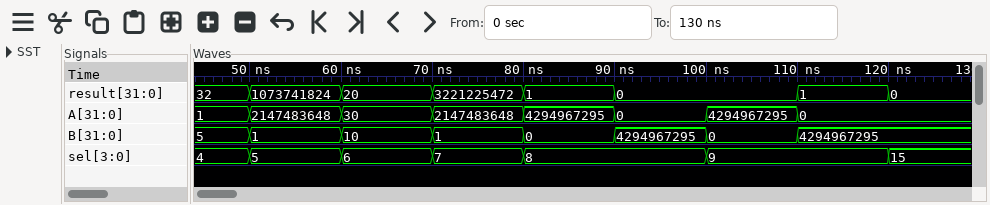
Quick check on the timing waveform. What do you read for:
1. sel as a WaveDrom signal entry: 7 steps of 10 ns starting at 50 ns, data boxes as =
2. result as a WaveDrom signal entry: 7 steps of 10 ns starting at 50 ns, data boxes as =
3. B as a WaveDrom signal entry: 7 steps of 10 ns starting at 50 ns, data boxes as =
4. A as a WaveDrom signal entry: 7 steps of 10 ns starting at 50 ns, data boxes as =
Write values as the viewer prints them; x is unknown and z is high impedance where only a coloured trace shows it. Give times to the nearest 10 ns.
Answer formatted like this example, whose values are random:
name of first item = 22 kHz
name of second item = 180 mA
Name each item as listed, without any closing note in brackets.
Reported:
sel as a WaveDrom signal entry: 7 steps of 10 ns starting at 50 ns, data boxes as = = {name: 'sel', wave: '====.=.', data: '5 6 7 8 9'}
result as a WaveDrom signal entry: 7 steps of 10 ns starting at 50 ns, data boxes as = = {name: 'result', wave: '=====.=', data: '1073741824 20 3221225472 1 0 1'}
B as a WaveDrom signal entry: 7 steps of 10 ns starting at 50 ns, data boxes as = = {name: 'B', wave: '=======', data: '1 10 1 0 4294967295 0 4294967295'}
A as a WaveDrom signal entry: 7 steps of 10 ns starting at 50 ns, data boxes as = = {name: 'A', wave: '=======', data: '2147483648 30 2147483648 4294967295 0 4294967295 0'}
